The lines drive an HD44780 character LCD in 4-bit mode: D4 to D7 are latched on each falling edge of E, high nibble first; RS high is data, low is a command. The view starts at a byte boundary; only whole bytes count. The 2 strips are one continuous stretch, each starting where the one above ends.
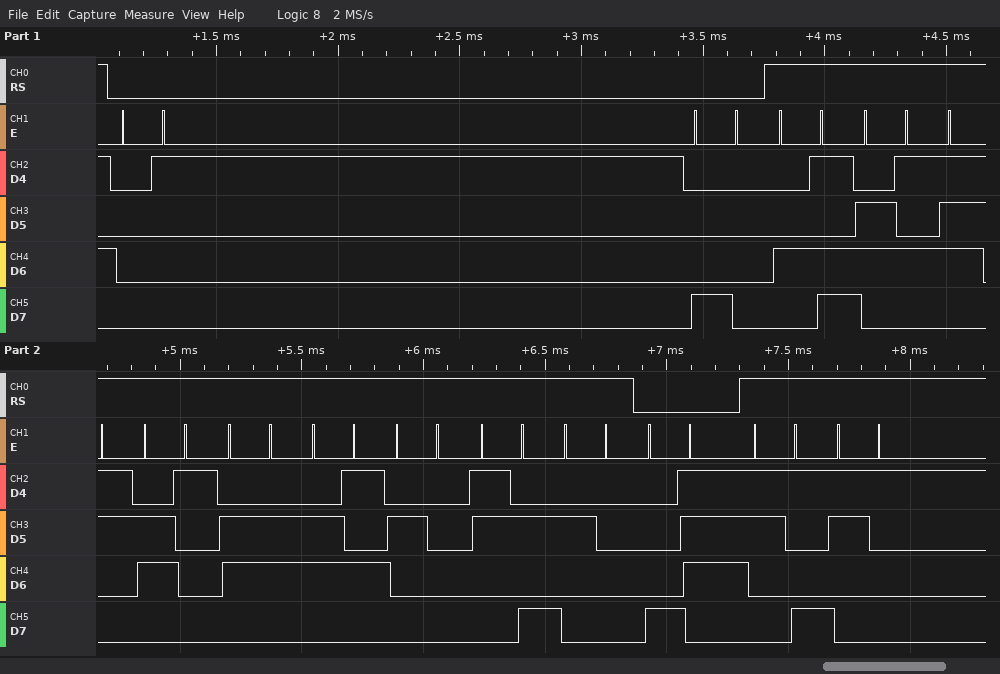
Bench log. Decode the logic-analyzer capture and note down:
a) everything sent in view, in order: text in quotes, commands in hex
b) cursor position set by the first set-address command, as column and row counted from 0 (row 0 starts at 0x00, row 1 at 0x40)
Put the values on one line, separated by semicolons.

0x01 0x80 "Mesafe : " 0x87 "91"; column 0, row 0
